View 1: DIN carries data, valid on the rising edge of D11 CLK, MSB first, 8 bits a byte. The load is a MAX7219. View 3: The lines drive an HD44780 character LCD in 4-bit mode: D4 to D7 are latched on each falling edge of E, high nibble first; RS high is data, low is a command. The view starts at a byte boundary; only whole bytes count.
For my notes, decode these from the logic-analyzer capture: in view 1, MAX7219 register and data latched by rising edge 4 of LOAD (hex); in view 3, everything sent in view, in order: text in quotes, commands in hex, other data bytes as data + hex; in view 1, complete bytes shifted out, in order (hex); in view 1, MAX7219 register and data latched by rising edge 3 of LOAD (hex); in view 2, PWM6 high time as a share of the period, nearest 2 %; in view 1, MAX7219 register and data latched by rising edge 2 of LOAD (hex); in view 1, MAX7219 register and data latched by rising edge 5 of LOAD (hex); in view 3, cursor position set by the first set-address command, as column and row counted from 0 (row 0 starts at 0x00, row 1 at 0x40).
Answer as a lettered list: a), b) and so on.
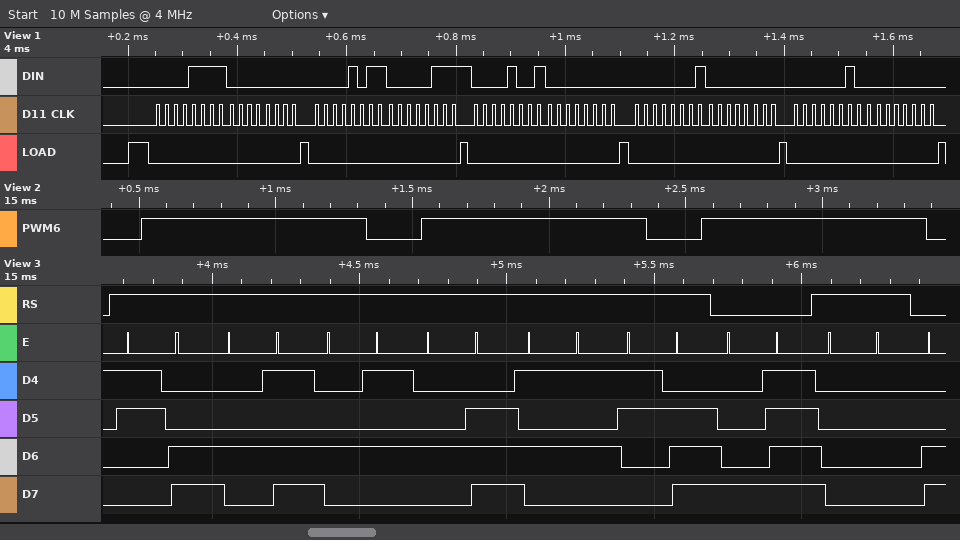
a) register 0x9, data 0x00
b) "<MENU>" 0x8F data 00
c) 0F 00 0B 07 09 00 01 00 02 00
d) register 0xB, data 0x07
e) 80 %
f) register 0xF, data 0x00
g) register 0x1, data 0x00
h) column 15, row 0
